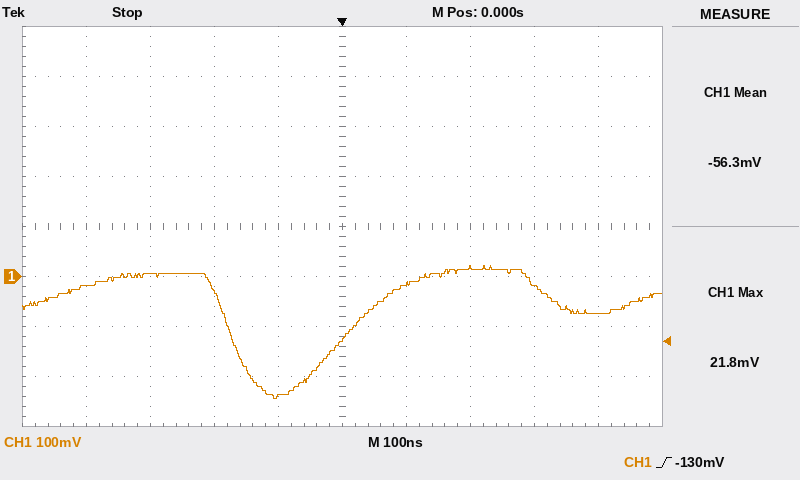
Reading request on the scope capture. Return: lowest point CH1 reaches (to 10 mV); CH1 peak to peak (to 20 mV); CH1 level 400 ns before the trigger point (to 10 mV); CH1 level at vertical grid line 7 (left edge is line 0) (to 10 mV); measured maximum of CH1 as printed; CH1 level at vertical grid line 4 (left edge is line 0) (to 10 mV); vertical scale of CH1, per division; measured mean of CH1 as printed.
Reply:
-240 mV
260 mV
-20 mV
20 mV
21.8 mV
-240 mV
100 mV
-56.3 mV
